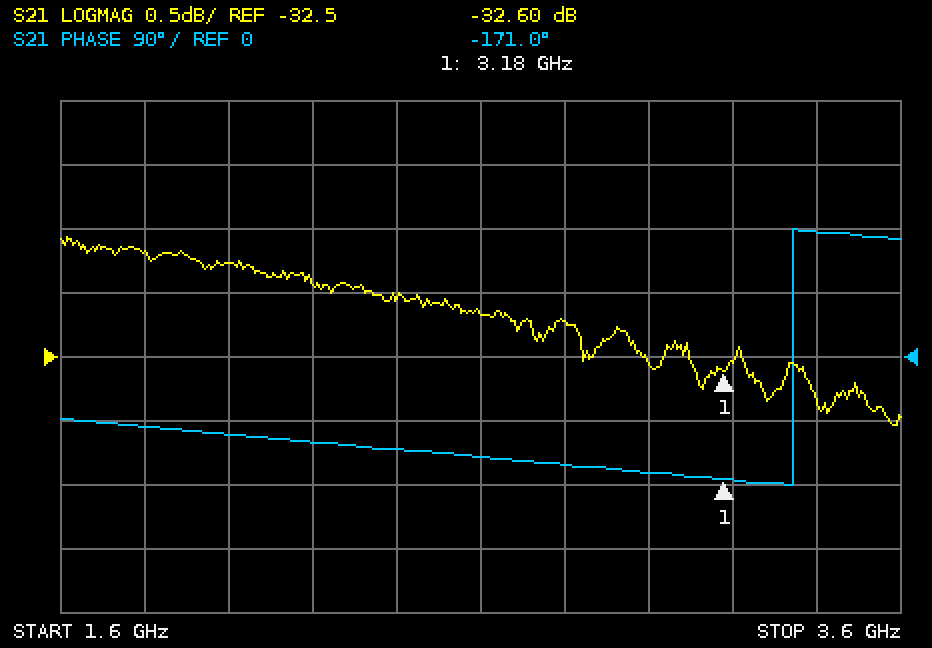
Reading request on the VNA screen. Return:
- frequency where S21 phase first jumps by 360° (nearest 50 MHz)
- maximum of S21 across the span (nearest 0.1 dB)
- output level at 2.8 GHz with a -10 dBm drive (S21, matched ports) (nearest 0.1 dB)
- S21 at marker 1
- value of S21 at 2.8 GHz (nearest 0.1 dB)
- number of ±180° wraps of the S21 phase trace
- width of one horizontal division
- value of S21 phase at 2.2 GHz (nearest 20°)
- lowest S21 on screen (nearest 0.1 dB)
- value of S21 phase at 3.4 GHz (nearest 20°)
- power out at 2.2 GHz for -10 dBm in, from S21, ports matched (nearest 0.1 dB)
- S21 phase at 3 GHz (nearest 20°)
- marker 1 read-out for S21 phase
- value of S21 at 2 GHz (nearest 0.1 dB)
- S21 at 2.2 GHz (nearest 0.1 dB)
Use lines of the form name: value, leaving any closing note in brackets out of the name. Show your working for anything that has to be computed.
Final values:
frequency where S21 phase first jumps by 360°: 3.35 GHz
maximum of S21 across the span: -31.6 dB
output level at 2.8 GHz with a -10 dBm drive (S21, matched ports): -10 dBm + (-32.2 dB) = -42.2 dBm
S21 at marker 1: -32.60 dB
value of S21 at 2.8 GHz: -32.2 dB
number of ±180° wraps of the S21 phase trace: 1
width of one horizontal division: 200 MHz
value of S21 phase at 2.2 GHz: -120°
lowest S21 on screen: -33.0 dB
value of S21 phase at 3.4 GHz: 180°
power out at 2.2 GHz for -10 dBm in, from S21, ports matched: -10 dBm + (-31.9 dB) = -41.9 dBm
S21 phase at 3 GHz: -160°
marker 1 read-out for S21 phase: -171.0°
value of S21 at 2 GHz: -31.8 dB
S21 at 2.2 GHz: -31.9 dB
